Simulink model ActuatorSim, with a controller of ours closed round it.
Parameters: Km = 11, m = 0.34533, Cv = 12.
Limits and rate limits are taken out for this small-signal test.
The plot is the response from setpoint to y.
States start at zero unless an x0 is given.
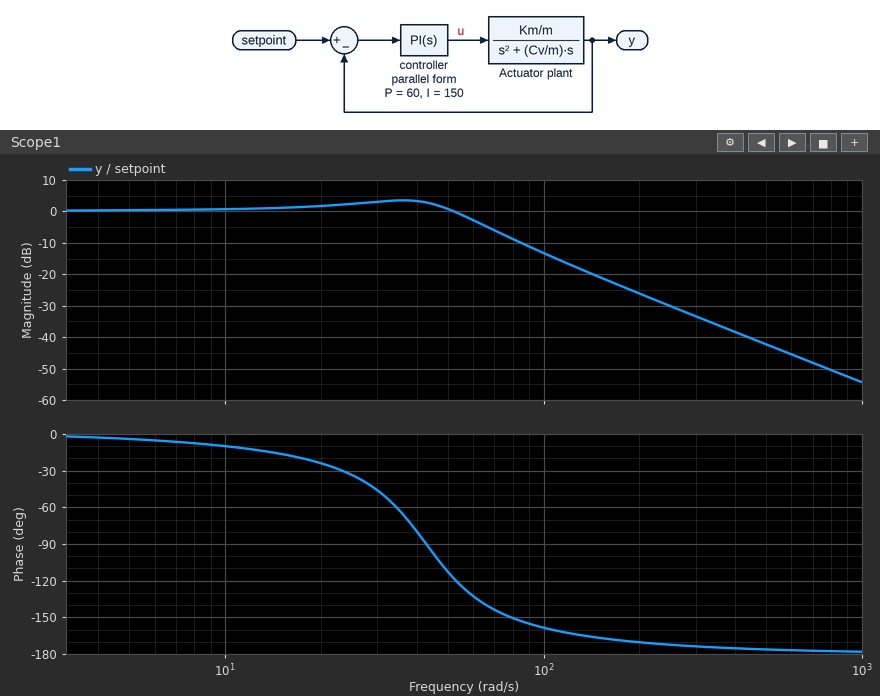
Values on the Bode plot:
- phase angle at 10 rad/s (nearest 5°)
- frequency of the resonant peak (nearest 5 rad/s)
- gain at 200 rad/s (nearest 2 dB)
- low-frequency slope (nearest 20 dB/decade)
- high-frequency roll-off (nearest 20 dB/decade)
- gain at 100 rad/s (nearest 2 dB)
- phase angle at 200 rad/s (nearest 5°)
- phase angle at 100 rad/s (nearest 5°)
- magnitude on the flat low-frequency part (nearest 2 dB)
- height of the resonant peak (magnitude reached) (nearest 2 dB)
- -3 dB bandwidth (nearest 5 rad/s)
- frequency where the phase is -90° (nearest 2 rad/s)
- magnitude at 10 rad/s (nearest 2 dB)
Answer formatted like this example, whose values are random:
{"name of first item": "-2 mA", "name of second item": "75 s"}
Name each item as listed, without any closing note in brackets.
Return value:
{"phase angle at 10 rad/s": "-10°", "frequency of the resonant peak": "35 rad/s", "gain at 200 rad/s": "-26 dB", "low-frequency slope": "0 dB/decade", "high-frequency roll-off": "-40 dB/decade", "gain at 100 rad/s": "-14 dB", "phase angle at 200 rad/s": "-170°", "phase angle at 100 rad/s": "-160°", "magnitude on the flat low-frequency part": "0 dB", "height of the resonant peak (magnitude reached)": "4 dB", "-3 dB bandwidth": "60 rad/s", "frequency where the phase is -90°": "42 rad/s", "magnitude at 10 rad/s": "0 dB"}
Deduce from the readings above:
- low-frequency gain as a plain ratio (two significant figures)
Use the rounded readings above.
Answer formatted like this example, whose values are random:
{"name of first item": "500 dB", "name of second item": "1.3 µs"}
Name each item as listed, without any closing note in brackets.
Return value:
{"low-frequency gain as a plain ratio": "1.0"}
